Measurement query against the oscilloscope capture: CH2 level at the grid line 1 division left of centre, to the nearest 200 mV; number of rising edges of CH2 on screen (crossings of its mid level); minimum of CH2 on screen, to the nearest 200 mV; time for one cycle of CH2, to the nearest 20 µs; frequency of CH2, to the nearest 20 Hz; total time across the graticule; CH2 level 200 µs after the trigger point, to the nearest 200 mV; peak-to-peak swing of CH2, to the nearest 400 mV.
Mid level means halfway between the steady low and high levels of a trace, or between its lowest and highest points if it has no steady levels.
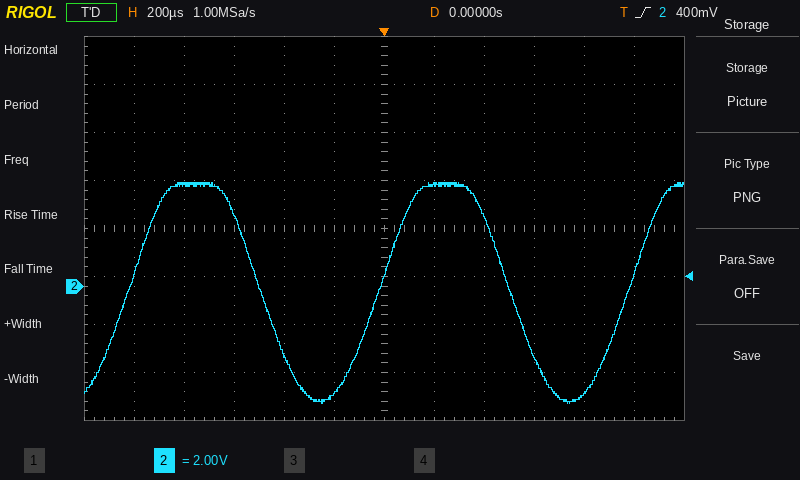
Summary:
-4.4 V
3
-4.8 V
1.00 ms
1.00 kHz
2.4 ms
4.2 V
9.2 V
